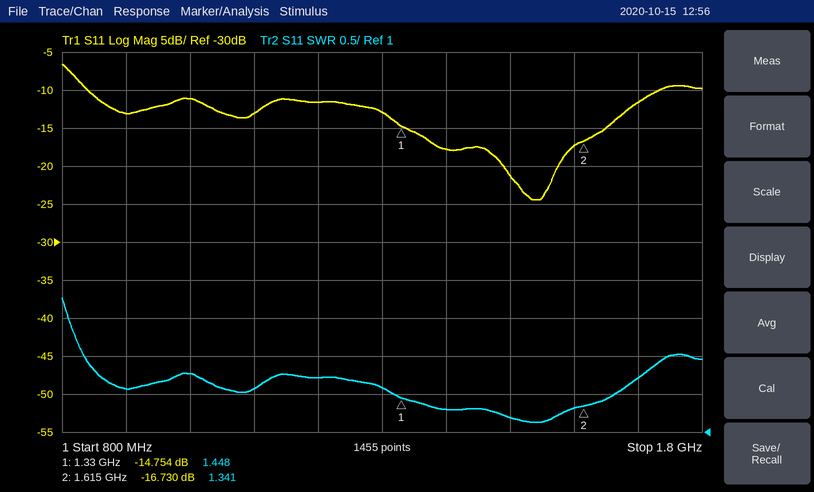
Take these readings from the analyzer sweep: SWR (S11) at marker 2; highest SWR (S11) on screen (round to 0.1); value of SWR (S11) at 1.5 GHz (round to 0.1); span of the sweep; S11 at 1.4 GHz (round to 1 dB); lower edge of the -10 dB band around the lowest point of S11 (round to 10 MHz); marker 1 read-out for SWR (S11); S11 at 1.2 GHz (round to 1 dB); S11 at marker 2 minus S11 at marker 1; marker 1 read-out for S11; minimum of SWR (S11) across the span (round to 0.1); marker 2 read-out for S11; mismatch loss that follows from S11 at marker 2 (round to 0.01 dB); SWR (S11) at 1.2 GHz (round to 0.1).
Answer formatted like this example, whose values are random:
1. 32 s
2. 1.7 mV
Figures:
1. 1.341
2. 2.8
3. 1.2
4. 1 GHz
5. -18 dB
6. 840 MHz
7. 1.448
8. -12 dB
9. -1.976 dB
10. -14.754 dB
11. 1.1
12. -16.730 dB
13. 0.09 dB
14. 1.7
